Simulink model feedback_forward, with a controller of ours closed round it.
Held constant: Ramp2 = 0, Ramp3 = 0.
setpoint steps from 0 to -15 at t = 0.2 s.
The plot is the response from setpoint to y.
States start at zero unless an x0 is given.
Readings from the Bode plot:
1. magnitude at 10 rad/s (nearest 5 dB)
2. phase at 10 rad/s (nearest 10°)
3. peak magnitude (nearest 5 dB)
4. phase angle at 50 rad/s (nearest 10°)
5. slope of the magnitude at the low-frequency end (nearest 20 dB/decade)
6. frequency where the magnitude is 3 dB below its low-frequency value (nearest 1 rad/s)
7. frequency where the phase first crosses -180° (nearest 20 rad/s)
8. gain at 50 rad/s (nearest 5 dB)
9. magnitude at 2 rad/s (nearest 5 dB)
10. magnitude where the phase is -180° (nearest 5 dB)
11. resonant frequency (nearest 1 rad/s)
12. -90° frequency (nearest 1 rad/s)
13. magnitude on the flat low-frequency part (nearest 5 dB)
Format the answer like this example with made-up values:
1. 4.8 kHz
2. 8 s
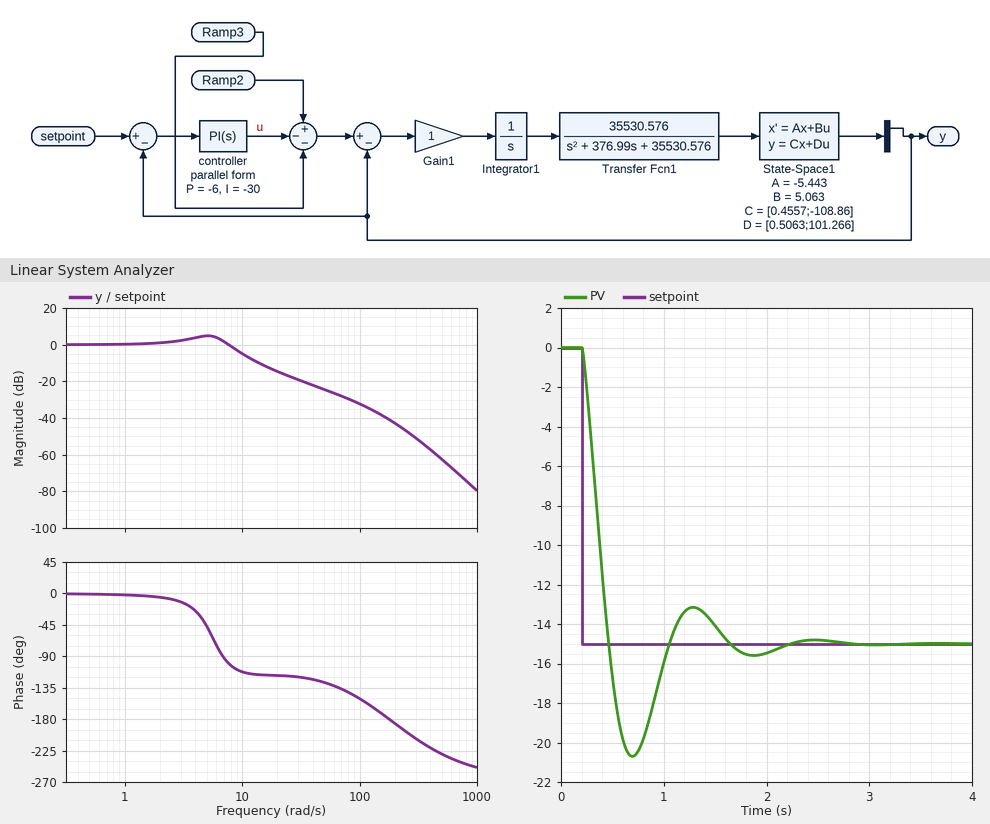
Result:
1. -5 dB
2. -110°
3. 5 dB
4. -130°
5. 0 dB/decade
6. 9 rad/s
7. 180 rad/s
8. -25 dB
9. 0 dB
10. -40 dB
11. 5 rad/s
12. 7 rad/s
13. 0 dB
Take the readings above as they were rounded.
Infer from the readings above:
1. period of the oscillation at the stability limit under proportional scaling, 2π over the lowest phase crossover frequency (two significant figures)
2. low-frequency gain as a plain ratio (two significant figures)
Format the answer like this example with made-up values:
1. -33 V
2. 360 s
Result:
1. 0.035 s
2. 1.0
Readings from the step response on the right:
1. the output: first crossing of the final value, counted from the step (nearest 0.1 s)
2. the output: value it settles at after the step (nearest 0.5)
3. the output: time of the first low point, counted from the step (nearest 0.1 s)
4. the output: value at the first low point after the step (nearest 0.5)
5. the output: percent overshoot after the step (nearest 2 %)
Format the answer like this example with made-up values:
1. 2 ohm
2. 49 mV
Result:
1. 0.3 s
2. -15.0
3. 0.5 s
4. -20.5
5. 38 %
